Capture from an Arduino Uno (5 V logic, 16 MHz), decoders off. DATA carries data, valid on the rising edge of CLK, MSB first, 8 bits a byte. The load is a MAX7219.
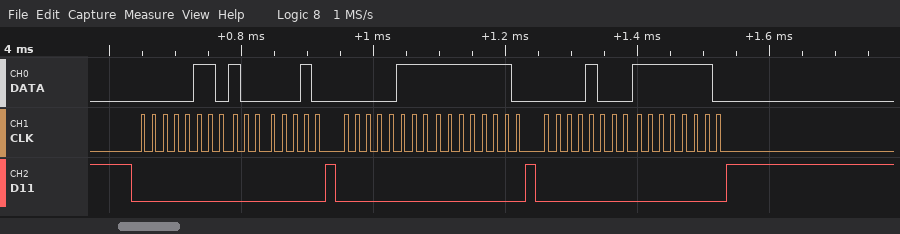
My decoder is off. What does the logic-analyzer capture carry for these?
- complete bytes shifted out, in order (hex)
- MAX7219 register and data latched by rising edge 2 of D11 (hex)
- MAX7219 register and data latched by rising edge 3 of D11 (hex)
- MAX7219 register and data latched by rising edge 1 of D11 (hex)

0x06 0x82 0x07 0xFE 0x08 0xFE
register 0x7, data 0xFE
register 0x8, data 0xFE
register 0x6, data 0x82
